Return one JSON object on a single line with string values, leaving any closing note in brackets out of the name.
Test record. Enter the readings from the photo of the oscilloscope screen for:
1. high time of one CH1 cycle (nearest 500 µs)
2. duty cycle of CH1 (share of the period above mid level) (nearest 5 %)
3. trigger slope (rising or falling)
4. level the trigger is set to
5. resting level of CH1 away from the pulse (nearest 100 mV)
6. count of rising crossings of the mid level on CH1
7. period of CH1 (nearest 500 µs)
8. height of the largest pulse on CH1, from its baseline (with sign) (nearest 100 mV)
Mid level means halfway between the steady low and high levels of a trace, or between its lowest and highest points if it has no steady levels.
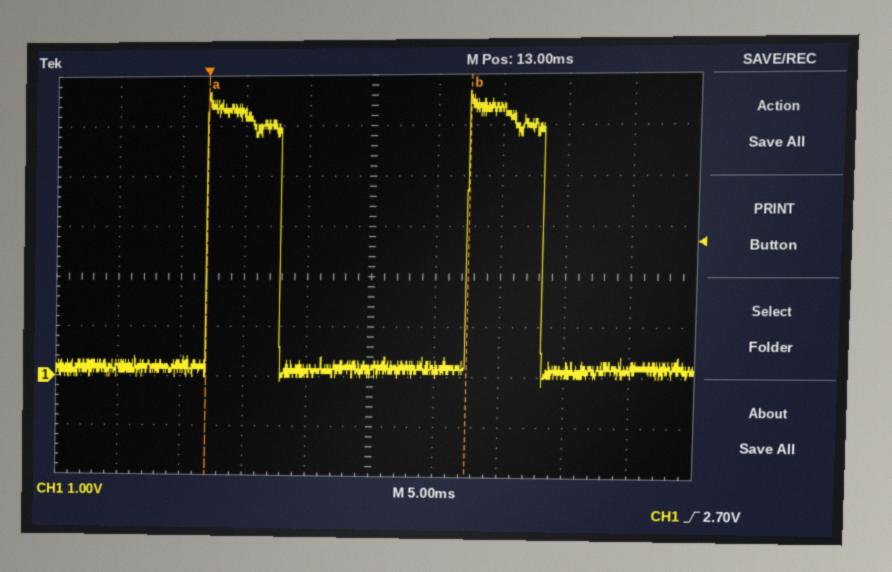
{"high time of one CH1 cycle": "6.0 ms", "duty cycle of CH1 (share of the period above mid level)": "30 %", "trigger slope": "rising", "level the trigger is set to": "2.70 V", "resting level of CH1 away from the pulse": "200 mV", "count of rising crossings of the mid level on CH1": "2", "period of CH1": "20.5 ms", "height of the largest pulse on CH1, from its baseline (with sign)": "+5.5 V"}
